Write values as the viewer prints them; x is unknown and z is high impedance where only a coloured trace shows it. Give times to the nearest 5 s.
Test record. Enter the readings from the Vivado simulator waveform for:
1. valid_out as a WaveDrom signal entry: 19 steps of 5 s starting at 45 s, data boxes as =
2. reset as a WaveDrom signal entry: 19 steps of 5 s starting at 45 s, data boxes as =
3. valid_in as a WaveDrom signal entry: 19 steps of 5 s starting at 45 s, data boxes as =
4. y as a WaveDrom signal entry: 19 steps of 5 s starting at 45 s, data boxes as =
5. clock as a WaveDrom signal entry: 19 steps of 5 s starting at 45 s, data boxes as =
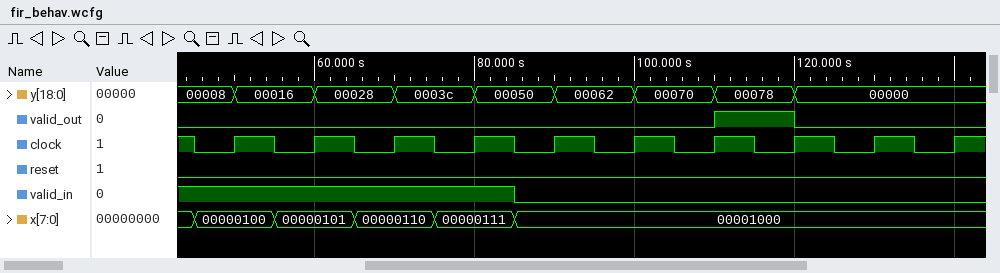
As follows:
{name: 'valid_out', wave: '0............1.0...'}
{name: 'reset', wave: '0..................'}
{name: 'valid_in', wave: '1.......0..........'}
{name: 'y', wave: '==.=.=.=.=.=.=.=...', data: '00008 00016 00028 0003c 00050 00062 00070 00078 00000'}
{name: 'clock', wave: '0101010101010101010'}
